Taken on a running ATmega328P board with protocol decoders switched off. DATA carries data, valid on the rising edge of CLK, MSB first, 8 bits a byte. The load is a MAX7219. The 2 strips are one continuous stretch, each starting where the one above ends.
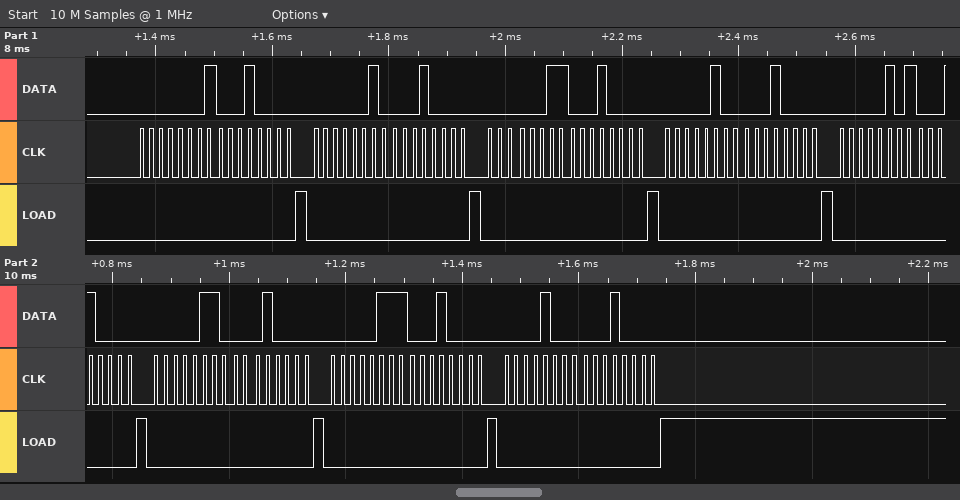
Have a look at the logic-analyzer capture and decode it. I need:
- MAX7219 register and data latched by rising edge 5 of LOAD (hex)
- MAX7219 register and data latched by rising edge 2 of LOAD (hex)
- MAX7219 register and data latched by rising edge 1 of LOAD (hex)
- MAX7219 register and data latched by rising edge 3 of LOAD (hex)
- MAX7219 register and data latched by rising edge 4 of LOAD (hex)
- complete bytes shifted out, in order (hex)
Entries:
register 0x5, data 0x10
register 0x2, data 0x10
register 0x1, data 0x10
register 0x3, data 0x10
register 0x4, data 0x10
01 10 02 10 03 10 04 10 05 10 06 10 07 10 08 10
